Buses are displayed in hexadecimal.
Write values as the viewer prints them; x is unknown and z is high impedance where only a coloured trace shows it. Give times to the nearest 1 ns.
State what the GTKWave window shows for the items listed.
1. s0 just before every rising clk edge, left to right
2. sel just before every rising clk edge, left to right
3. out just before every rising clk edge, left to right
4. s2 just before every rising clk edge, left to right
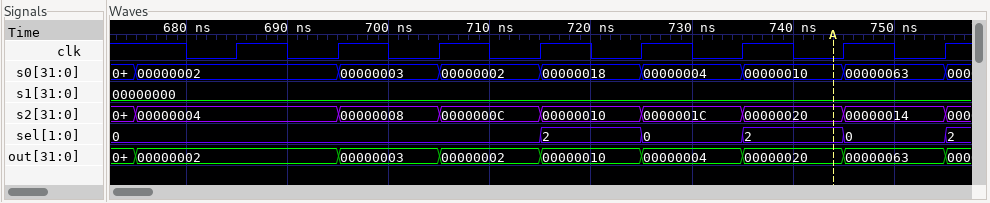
00000002, 00000002, 00000003, 00000002, 00000018, 00000004, 00000010, 00000063
0, 0, 0, 0, 2, 0, 2, 0
00000002, 00000002, 00000003, 00000002, 00000010, 00000004, 00000020, 00000063
00000004, 00000004, 00000008, 0000000C, 00000010, 0000001C, 00000020, 00000014
